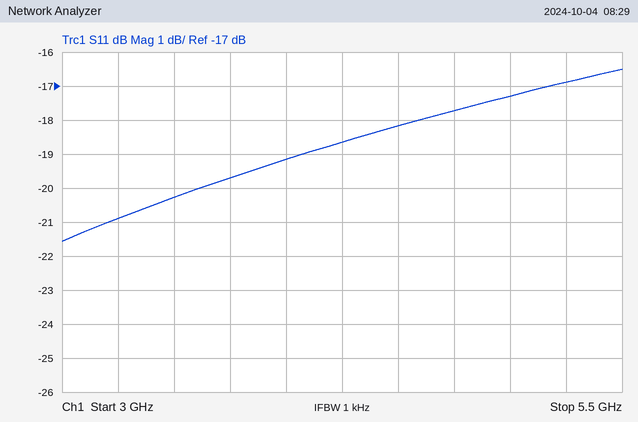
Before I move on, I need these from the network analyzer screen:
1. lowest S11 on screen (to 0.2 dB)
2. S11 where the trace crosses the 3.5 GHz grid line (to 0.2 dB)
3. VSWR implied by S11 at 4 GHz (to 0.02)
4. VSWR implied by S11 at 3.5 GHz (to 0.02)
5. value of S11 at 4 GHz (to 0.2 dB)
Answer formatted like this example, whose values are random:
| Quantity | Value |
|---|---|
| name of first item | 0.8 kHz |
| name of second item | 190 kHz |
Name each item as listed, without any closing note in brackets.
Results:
| Quantity | Value |
|---|---|
| lowest S11 on screen | -21.6 dB |
| S11 where the trace crosses the 3.5 GHz grid line | -20.2 dB |
| VSWR implied by S11 at 4 GHz | 1.24 |
| VSWR implied by S11 at 3.5 GHz | 1.22 |
| value of S11 at 4 GHz | -19.2 dB |
